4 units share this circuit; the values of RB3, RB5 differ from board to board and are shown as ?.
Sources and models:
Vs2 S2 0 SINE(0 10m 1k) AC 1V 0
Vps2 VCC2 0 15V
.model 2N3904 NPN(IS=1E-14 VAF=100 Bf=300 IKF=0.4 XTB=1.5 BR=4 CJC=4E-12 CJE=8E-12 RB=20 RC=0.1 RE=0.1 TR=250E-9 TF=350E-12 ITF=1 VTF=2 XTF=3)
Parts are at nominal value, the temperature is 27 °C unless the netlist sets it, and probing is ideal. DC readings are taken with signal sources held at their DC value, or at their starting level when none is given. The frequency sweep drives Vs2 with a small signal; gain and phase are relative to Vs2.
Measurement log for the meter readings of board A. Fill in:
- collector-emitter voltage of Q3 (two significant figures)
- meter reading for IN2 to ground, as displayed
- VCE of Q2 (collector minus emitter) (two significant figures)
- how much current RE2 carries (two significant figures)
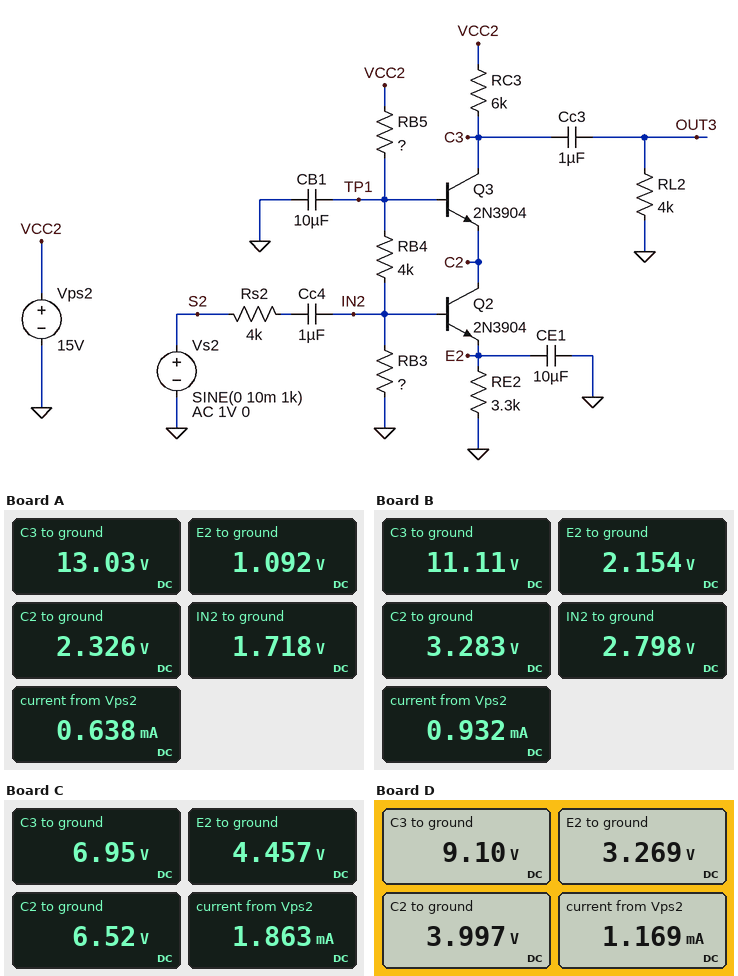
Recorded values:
11 V
1.718 V
1.2 V
330 µA
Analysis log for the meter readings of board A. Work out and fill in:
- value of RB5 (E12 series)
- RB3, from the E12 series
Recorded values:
39 kΩ
5.6 kΩ
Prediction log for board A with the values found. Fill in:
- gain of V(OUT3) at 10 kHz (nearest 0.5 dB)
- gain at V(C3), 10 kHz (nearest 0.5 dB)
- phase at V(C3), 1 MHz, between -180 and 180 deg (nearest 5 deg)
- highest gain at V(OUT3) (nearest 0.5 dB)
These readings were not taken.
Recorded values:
20.5 dB
20.5 dB
165 deg
20.5 dB
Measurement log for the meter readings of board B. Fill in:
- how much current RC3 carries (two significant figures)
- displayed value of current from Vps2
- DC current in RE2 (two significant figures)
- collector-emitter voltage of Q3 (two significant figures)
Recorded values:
650 µA
0.932 mA
650 µA
7.8 V
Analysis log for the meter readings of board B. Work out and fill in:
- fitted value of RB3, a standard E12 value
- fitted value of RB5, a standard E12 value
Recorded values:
10 kΩ
39 kΩ
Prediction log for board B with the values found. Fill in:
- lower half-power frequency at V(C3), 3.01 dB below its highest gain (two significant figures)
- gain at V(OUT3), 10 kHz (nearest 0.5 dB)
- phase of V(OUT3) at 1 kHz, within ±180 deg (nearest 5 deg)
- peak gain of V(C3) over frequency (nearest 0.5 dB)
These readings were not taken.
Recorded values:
360 Hz
27.0 dB
-160 deg
27.0 dB
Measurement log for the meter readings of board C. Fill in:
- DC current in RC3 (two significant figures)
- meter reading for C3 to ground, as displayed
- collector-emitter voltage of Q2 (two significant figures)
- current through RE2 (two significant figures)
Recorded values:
1.3 mA
6.95 V
2.1 V
1.4 mA
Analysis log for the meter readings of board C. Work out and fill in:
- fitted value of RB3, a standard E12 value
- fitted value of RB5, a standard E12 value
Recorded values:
10 kΩ
15 kΩ
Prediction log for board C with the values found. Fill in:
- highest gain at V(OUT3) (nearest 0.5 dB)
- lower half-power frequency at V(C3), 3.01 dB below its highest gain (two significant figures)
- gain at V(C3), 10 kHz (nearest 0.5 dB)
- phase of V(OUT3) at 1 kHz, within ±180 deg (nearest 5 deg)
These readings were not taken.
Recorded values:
32.0 dB
650 Hz
32.0 dB
-145 deg
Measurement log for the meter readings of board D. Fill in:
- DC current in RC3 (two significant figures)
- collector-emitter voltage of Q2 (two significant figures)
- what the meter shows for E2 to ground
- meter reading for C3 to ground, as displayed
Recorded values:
980 µA
730 mV
3.269 V
9.10 V
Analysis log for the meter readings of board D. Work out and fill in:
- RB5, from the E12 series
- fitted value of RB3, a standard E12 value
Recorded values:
56 kΩ
22 kΩ
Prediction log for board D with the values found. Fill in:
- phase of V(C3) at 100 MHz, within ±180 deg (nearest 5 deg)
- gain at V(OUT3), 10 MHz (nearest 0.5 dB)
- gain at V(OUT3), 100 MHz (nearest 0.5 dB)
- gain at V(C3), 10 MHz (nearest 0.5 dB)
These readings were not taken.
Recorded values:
-10 deg
19.5 dB
-11.5 dB
19.5 dB
